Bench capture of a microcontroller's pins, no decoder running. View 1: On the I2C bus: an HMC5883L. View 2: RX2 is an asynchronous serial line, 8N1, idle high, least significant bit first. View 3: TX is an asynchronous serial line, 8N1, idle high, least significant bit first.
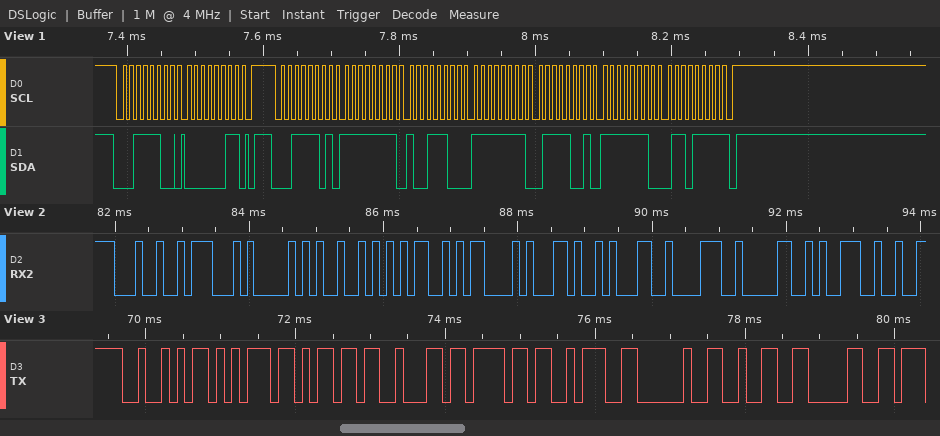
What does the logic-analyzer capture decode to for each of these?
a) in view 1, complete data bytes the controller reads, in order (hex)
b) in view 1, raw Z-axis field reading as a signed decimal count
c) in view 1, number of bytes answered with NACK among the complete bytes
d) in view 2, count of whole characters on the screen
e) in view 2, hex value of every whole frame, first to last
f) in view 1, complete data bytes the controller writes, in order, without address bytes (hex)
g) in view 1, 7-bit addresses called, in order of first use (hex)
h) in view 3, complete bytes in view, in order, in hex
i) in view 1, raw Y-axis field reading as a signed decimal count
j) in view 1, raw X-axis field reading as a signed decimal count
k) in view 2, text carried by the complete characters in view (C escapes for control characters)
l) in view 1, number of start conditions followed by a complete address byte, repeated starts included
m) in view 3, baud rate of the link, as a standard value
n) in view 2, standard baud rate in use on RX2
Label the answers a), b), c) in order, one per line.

a) FF 9C FF 79 FE 6F
b) -135
c) 1
d) 11
e) 24 47 50 52 4D 43 2C 31 38 30 39
f) 03
g) 0x1E
h) 0x52 0x75 0x6D 0x62 0x6F 0x3A 0x20 0x32 0x30
i) -401
j) -100
k) "$GPRMC,1809"
l) 2
m) 9600 baud
n) 9600 baud
